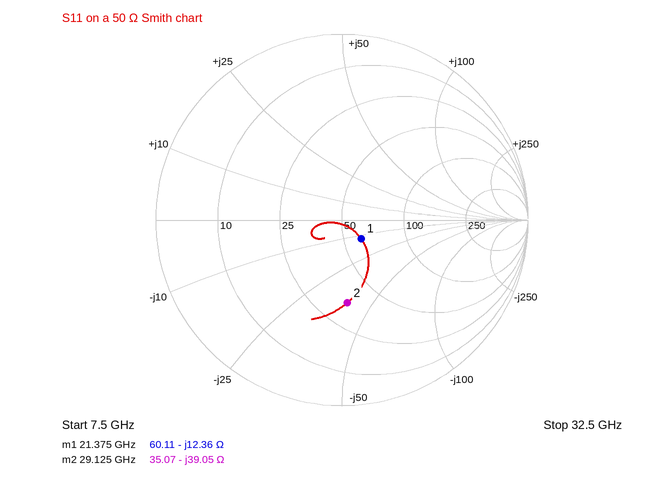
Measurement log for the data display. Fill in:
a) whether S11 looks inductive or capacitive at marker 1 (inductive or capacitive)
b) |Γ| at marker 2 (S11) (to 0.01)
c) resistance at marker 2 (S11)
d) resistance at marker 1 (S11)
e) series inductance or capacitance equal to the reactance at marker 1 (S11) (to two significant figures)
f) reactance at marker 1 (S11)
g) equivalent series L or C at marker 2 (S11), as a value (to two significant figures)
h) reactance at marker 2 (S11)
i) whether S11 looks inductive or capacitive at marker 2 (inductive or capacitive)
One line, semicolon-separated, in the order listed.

capacitive; 0.45; 35.07 Ω; 60.11 Ω; 600 fF; -12.36 Ω; 140 fF; -39.05 Ω; capacitive
